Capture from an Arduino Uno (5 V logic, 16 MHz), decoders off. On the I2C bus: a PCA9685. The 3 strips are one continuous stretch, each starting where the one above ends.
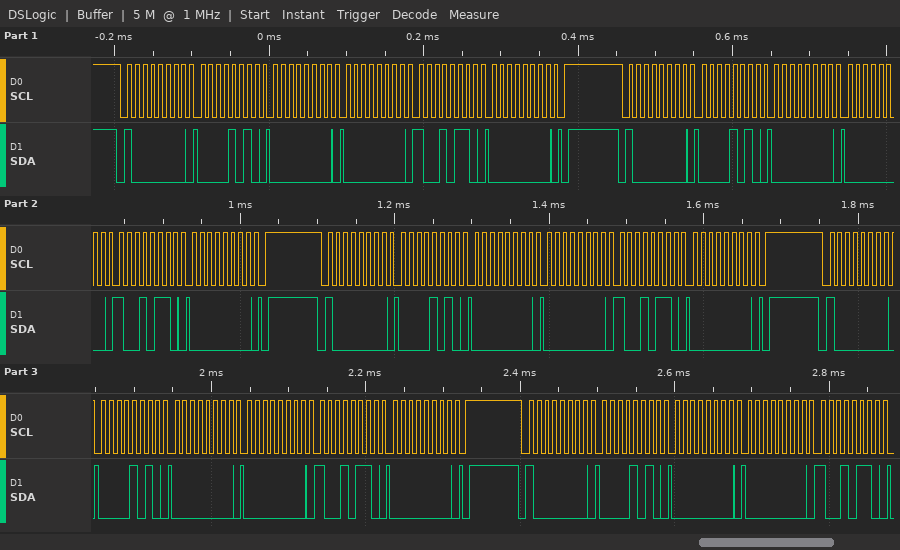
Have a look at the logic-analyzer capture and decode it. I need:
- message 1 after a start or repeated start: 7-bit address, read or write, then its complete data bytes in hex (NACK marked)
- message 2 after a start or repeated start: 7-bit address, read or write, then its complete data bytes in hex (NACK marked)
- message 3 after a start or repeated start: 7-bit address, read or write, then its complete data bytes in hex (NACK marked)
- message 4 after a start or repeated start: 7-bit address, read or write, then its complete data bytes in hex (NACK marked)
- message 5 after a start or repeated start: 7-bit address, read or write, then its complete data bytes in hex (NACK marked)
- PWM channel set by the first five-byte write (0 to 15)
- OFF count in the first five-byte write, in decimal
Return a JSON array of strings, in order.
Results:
["0x40 write: 0A 00 00 96 00", "0x40 write: 0A 00 00 96 00", "0x40 write: 0A 00 00 96 00", "0x40 write: 0A 00 00 96 00", "0x40 write: 0A 00 00 96", "1", "150"]
